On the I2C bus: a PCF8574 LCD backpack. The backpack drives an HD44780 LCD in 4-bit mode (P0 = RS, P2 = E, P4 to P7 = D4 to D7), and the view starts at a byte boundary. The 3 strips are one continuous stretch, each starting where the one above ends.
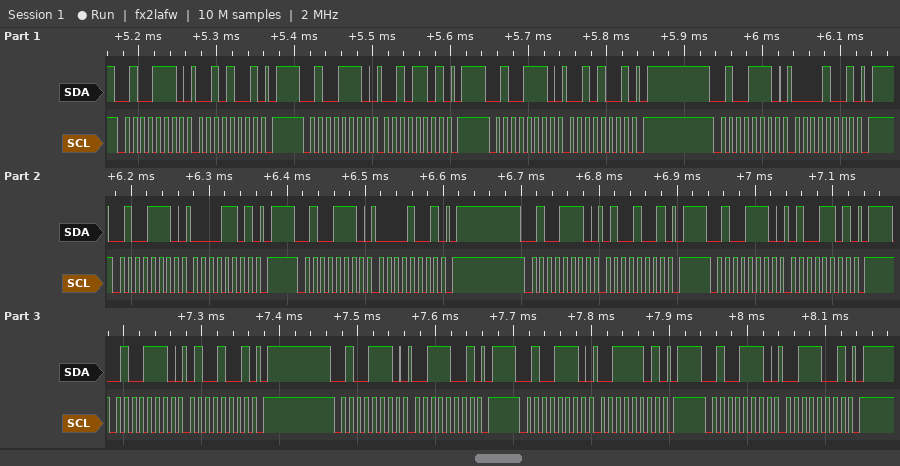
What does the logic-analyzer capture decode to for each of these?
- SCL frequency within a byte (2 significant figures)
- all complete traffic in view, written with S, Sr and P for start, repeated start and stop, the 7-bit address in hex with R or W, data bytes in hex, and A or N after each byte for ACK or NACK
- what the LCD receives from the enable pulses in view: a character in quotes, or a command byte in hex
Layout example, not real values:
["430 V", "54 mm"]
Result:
["100 kHz", "S 27W A 29 A P S 27W A 2D A P S 27W A 29 A P S 27W A 09 A P S 27W A 0D A P S 27W A 09 A P S 27W A 49 A P S 27W A 4D A P S 27W A 49 A P S 27W A 39 A P S 27W A 3D A P S 27W A 39 A P", "' ' 'C'"]
